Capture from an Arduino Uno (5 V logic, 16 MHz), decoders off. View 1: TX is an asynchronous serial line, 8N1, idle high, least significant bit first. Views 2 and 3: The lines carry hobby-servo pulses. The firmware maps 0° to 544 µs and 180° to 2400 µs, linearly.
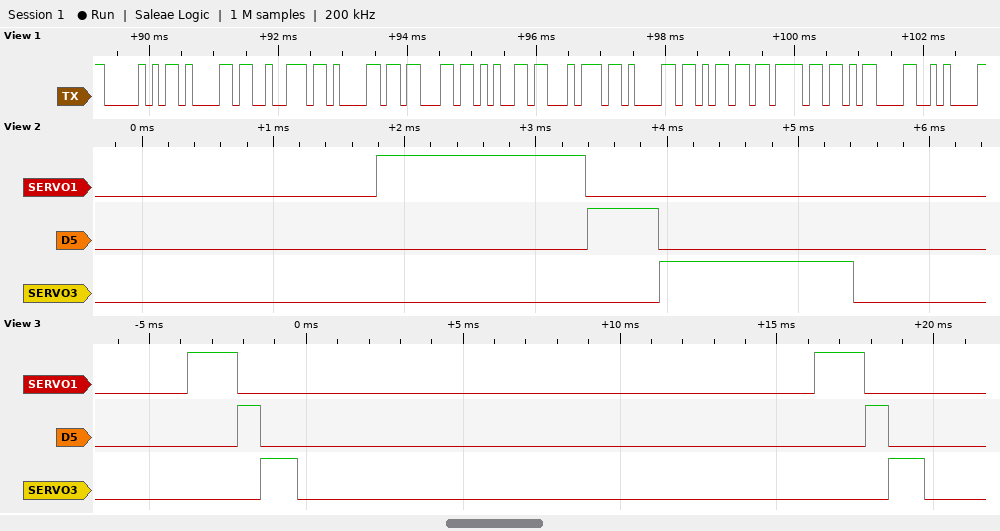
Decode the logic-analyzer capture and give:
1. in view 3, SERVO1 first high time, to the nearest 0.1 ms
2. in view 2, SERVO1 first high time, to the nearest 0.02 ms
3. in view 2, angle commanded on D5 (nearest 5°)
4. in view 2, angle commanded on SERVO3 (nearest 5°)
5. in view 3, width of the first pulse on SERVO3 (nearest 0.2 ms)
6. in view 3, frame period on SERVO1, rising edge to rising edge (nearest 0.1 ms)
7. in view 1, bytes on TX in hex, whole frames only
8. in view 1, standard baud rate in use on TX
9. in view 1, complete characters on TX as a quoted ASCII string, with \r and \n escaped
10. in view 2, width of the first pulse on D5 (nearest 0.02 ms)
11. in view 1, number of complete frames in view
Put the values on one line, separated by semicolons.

1.6 ms; 1.60 ms; 0°; 90°; 1.2 ms; 20.0 ms; 0x50 0x61 0x72 0x61 0x63 0x65 0x74 0x61 0x6D 0x6F 0x0D 0x0A; 9600 baud; "Paracetamo\r\n"; 0.54 ms; 12
